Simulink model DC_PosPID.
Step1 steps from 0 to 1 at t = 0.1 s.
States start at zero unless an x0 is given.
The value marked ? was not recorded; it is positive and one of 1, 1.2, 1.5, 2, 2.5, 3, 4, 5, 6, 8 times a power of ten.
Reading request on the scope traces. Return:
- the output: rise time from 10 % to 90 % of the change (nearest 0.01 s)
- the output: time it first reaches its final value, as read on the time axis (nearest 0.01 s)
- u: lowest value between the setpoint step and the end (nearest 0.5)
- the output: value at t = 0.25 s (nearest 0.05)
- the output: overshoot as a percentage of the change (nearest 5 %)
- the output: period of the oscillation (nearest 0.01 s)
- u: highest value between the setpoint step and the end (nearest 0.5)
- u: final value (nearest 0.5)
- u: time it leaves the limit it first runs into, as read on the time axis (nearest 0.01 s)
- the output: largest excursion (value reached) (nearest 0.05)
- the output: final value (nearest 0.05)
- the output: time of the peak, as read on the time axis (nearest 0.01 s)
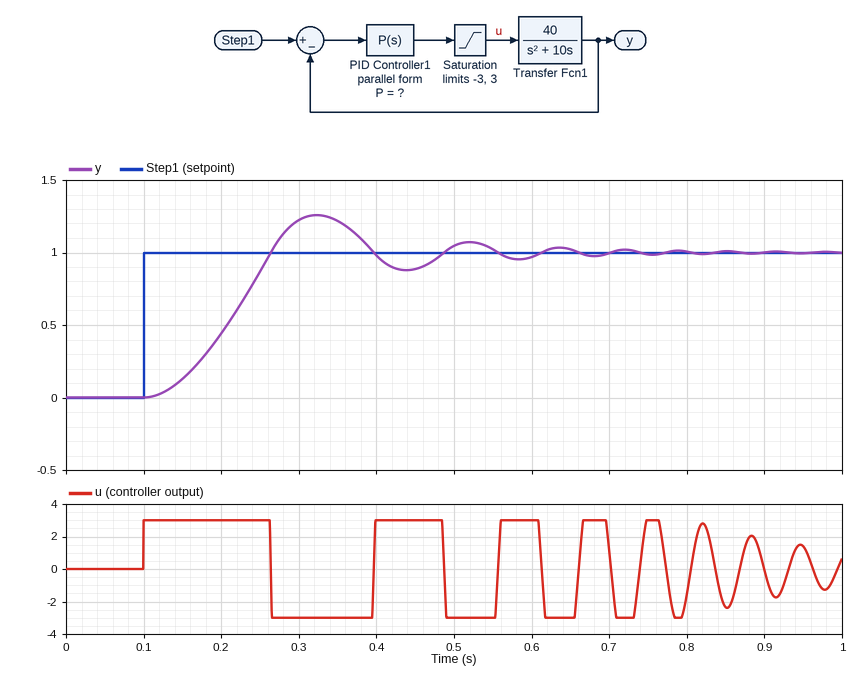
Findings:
0.11 s
0.26 s
-3.0
0.85
25 %
0.20 s
3.0
0.0
0.26 s
1.25
1.00
0.32 s
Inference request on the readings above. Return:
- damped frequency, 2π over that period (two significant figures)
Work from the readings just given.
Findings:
31 rad/s
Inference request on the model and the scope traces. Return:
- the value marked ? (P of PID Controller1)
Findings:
250
